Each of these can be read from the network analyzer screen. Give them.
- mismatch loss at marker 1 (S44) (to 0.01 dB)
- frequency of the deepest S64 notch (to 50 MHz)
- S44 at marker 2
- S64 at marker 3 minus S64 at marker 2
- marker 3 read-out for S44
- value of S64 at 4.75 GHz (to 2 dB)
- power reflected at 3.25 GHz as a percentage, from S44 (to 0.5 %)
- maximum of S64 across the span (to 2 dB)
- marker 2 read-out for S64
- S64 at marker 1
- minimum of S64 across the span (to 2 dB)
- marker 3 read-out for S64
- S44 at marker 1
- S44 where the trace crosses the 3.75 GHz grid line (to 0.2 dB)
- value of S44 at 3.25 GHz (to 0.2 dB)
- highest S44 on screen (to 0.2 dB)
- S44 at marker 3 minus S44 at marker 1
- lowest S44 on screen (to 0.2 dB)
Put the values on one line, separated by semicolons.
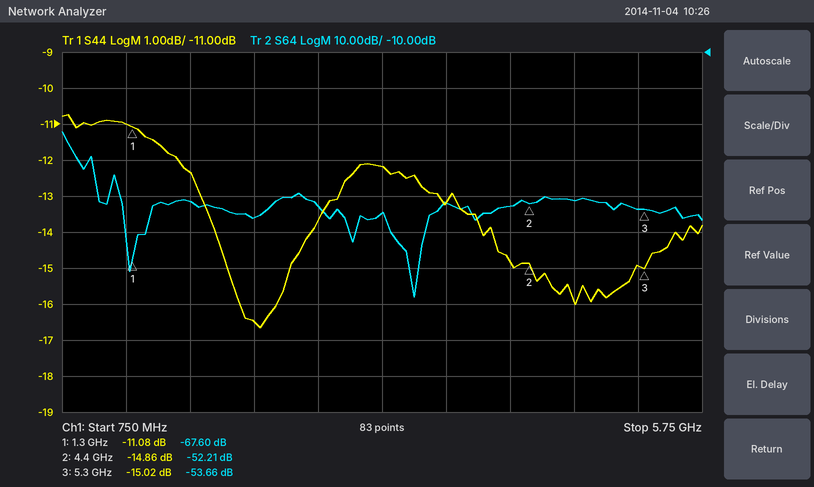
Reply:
0.35 dB; 3.50 GHz; -14.86 dB; -1.45 dB; -15.02 dB; -52 dB; 6.0 %; -32 dB; -52.21 dB; -67.60 dB; -78 dB; -53.66 dB; -11.08 dB; -13.2 dB; -12.2 dB; -10.8 dB; -3.94 dB; -16.6 dB
